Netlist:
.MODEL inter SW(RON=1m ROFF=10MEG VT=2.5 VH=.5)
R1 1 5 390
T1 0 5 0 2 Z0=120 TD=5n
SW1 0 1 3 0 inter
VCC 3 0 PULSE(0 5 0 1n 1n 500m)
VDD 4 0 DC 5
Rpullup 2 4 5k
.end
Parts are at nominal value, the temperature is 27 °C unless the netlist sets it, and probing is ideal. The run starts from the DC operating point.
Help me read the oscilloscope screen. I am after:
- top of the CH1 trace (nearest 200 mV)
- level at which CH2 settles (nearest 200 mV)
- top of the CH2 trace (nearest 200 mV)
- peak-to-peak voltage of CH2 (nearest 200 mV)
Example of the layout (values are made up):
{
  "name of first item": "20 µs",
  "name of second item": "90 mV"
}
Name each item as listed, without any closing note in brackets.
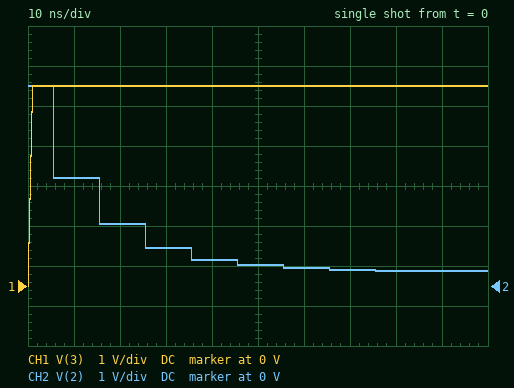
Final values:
{
  "top of the CH1 trace": "5.0 V",
  "level at which CH2 settles": "400 mV",
  "top of the CH2 trace": "5.0 V",
  "peak-to-peak voltage of CH2": "4.6 V"
}
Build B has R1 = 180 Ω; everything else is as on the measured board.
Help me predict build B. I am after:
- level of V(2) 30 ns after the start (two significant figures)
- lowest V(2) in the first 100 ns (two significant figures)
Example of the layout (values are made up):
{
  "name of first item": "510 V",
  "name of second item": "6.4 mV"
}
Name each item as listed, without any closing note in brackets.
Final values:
{
  "level of V(2) 30 ns after the start": "210 mV",
  "lowest V(2) in the first 100 ns": "170 mV"
}
